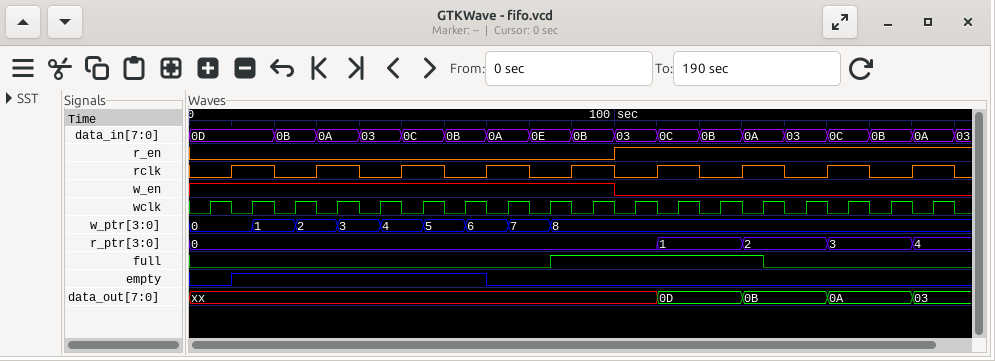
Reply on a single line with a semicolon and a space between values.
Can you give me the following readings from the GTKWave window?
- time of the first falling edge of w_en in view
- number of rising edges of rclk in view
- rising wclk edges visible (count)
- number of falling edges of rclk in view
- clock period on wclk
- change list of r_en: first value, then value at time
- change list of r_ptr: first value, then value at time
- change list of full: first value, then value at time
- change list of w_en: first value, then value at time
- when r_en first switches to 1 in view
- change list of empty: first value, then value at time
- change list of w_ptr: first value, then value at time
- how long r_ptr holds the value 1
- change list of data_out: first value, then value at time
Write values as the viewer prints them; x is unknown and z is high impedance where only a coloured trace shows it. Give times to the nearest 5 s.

100 s; 9; 18; 9; 10 s; 0, 1 at 100 s; 0, 1 at 110 s, 2 at 130 s, 3 at 150 s, 4 at 170 s; 0, 1 at 85 s, 0 at 135 s; 1, 0 at 100 s; 100 s; 0, 1 at 10 s, 0 at 70 s; 0, 1 at 15 s, 2 at 25 s, 3 at 35 s, 4 at 45 s, 5 at 55 s, 6 at 65 s, 7 at 75 s, 8 at 85 s; 20 s; xx, 0D at 110 s, 0B at 130 s, 0A at 150 s, 03 at 170 s
